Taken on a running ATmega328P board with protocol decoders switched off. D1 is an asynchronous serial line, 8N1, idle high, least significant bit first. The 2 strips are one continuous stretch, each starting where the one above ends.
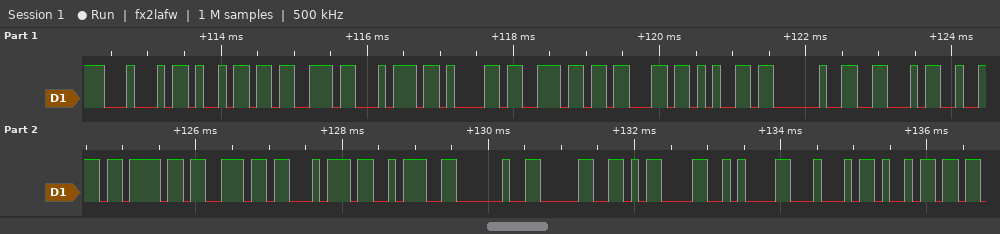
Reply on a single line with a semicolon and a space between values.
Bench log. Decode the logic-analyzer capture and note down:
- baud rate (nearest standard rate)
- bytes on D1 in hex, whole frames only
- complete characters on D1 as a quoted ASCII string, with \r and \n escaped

9600 baud; 44 69 73 74 61 6E 63 65 20 46 72 6F 6E 74 3A 20 30 0D 0A 44 69; "Distance Front: 0\r\nDi"
